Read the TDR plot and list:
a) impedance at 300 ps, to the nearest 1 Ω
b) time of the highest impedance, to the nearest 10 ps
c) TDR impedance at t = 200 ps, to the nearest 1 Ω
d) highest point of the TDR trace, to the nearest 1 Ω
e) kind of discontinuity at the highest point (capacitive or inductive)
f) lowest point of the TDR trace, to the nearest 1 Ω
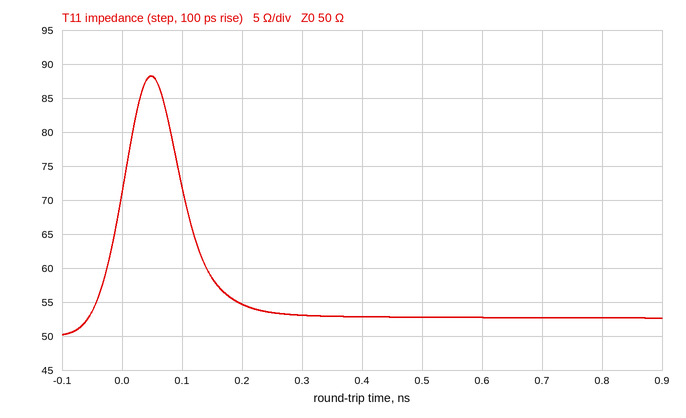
53 Ω
50 ps
55 Ω
88 Ω
inductive
50 Ω
